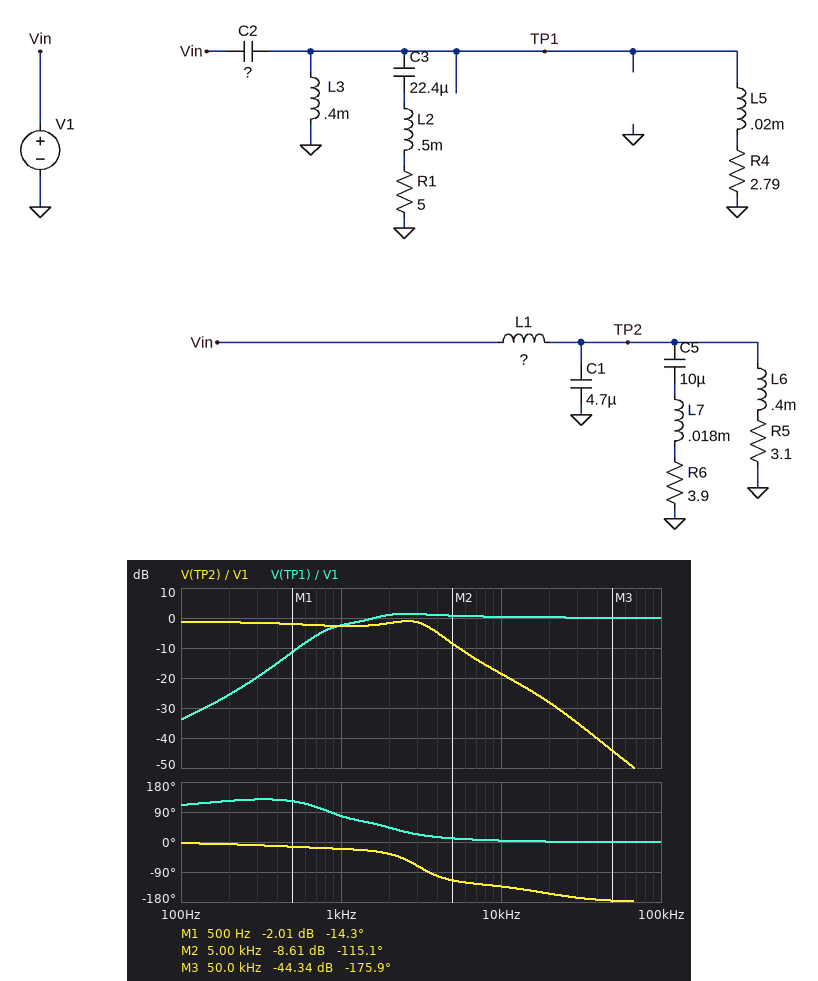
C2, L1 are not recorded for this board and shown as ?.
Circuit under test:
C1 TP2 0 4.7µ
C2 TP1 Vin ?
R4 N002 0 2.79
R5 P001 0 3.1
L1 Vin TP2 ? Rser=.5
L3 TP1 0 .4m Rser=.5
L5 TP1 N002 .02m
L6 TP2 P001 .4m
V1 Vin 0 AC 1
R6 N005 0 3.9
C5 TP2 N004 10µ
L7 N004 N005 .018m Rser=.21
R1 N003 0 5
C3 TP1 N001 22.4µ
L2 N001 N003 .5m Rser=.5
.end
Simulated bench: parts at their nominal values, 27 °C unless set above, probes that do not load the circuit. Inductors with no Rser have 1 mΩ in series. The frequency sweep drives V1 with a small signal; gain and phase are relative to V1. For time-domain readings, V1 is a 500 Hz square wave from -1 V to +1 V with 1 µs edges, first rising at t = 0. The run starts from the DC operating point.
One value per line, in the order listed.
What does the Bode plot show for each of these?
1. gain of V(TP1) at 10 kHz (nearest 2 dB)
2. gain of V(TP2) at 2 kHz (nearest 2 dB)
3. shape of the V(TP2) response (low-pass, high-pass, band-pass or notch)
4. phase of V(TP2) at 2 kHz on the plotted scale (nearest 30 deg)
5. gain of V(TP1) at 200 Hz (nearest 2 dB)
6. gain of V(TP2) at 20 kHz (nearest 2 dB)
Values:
0 dB
-2 dB
low-pass
-30 deg
-26 dB
-28 dB
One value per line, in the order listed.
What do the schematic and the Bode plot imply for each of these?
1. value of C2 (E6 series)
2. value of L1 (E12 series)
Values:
68 µF
390 µH
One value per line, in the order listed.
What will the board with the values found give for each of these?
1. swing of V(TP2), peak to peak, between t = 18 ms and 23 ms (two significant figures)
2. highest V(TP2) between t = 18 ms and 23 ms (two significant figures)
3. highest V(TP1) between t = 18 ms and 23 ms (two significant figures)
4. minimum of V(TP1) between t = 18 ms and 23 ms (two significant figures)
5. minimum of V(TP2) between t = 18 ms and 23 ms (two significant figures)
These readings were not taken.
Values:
1.8 V
880 mV
2.0 V
-2.0 V
-880 mV
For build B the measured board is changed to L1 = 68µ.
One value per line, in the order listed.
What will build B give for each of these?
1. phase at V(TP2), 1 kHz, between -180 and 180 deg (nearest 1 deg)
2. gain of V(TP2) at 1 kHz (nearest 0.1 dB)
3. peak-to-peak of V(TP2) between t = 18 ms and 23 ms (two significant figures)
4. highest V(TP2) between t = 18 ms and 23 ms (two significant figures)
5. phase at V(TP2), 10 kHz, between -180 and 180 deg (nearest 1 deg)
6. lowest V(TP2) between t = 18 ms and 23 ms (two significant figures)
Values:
-3 deg
-1.1 dB
2.7 V
1.3 V
-94 deg
-1.3 V
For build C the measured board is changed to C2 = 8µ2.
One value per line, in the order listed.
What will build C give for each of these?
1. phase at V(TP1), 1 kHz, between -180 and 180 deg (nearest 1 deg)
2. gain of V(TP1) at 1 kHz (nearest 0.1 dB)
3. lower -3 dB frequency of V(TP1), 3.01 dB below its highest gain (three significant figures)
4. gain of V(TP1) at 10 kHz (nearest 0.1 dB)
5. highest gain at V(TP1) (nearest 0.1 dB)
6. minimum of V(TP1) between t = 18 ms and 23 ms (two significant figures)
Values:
115 deg
-21.5 dB
6.38 kHz
1.5 dB
2.0 dB
-2.0 V
